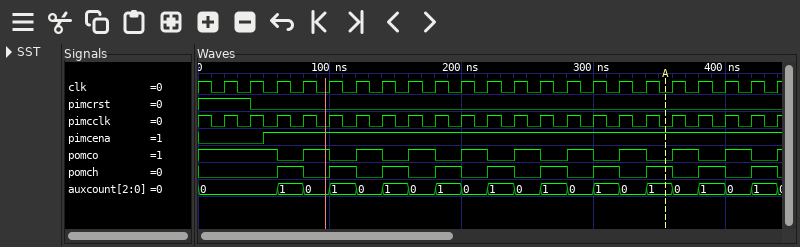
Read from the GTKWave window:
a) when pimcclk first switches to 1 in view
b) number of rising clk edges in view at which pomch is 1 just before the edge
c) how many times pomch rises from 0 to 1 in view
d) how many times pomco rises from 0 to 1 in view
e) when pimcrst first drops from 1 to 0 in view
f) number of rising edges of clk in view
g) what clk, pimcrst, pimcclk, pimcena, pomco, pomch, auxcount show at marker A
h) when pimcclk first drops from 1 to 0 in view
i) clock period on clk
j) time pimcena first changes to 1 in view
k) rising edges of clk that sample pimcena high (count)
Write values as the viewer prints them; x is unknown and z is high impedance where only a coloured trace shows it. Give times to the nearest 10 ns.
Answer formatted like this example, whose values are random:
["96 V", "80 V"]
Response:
["20 ns", "10", "10", "10", "40 ns", "22", "clk=0, pimcrst=0, pimcclk=0, pimcena=1, pomco=0, pomch=1, auxcount=1", "10 ns", "20 ns", "50 ns", "20"]
